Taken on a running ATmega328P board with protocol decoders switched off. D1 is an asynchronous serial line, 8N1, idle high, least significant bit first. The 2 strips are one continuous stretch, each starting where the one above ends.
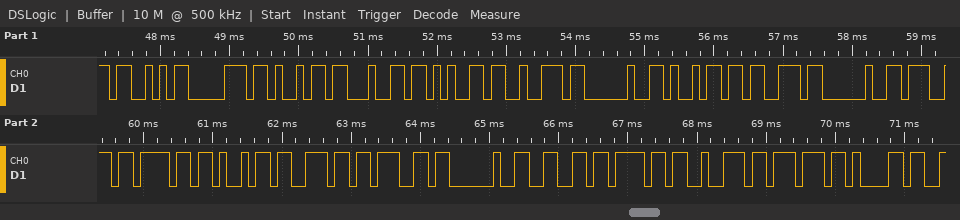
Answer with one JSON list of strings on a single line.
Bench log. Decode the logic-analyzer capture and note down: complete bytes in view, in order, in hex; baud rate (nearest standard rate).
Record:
["0x53 0x70 0x69 0x64 0x65 0x72 0x20 0x69 0x73 0x20 0x67 0x6F 0x69 0x6E 0x67 0x20 0x66 0x6F 0x72 0x77 0x61", "9600 baud"]
